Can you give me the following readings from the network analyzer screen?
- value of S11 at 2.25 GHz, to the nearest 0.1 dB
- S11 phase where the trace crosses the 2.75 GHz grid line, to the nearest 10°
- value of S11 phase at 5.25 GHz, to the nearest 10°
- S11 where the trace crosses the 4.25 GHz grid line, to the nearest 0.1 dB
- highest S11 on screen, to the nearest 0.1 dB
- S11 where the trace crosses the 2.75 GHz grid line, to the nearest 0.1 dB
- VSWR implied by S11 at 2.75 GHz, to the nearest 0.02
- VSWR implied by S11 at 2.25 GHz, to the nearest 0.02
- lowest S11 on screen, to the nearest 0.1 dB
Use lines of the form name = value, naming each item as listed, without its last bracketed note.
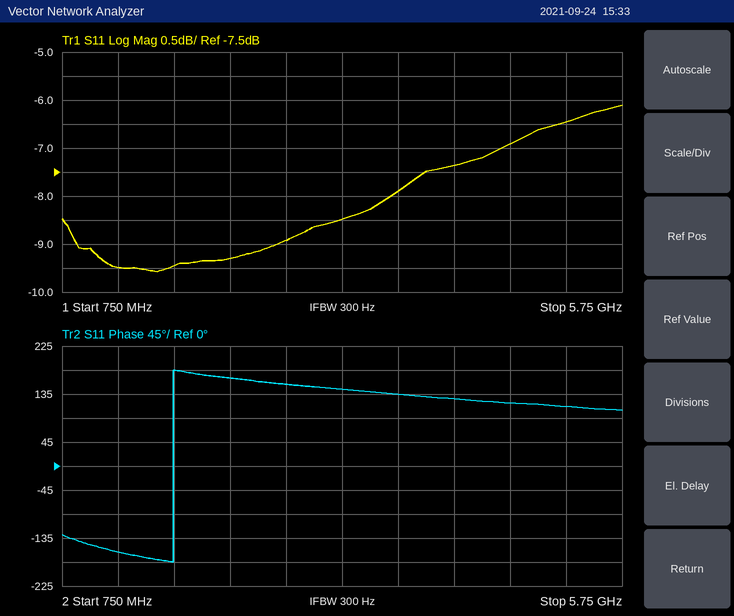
value of S11 at 2.25 GHz, to the nearest 0.1 dB = -9.3 dB
S11 phase where the trace crosses the 2.75 GHz grid line, to the nearest 10° = 150°
value of S11 phase at 5.25 GHz, to the nearest 10° = 110°
S11 where the trace crosses the 4.25 GHz grid line, to the nearest 0.1 dB = -7.4 dB
highest S11 on screen, to the nearest 0.1 dB = -6.1 dB
S11 where the trace crosses the 2.75 GHz grid line, to the nearest 0.1 dB = -8.9 dB
VSWR implied by S11 at 2.75 GHz, to the nearest 0.02 = 2.12
VSWR implied by S11 at 2.25 GHz, to the nearest 0.02 = 2.04
lowest S11 on screen, to the nearest 0.1 dB = -9.6 dB
